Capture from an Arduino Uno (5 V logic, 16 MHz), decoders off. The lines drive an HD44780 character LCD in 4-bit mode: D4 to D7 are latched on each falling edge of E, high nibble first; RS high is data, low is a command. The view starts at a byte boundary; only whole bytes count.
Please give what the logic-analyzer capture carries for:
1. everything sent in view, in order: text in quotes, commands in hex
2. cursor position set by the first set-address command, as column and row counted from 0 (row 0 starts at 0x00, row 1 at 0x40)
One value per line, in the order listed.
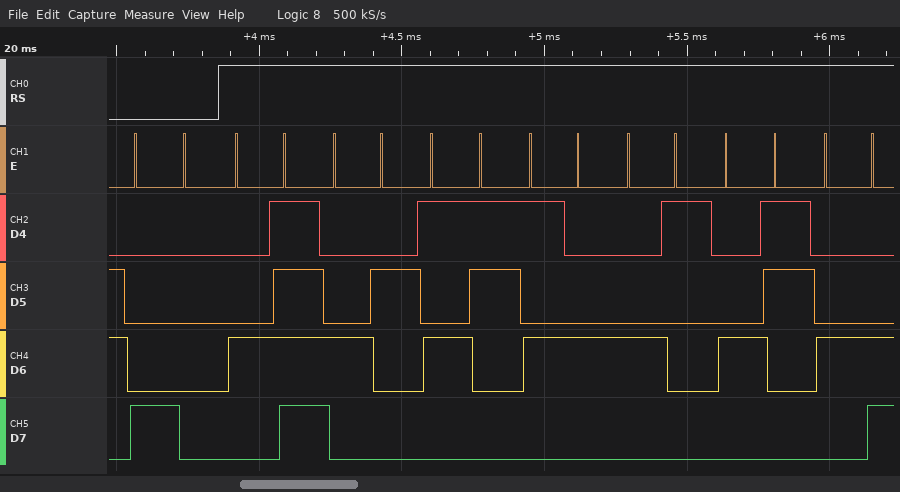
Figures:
0x80 "OBSTACL"
column 0, row 0
